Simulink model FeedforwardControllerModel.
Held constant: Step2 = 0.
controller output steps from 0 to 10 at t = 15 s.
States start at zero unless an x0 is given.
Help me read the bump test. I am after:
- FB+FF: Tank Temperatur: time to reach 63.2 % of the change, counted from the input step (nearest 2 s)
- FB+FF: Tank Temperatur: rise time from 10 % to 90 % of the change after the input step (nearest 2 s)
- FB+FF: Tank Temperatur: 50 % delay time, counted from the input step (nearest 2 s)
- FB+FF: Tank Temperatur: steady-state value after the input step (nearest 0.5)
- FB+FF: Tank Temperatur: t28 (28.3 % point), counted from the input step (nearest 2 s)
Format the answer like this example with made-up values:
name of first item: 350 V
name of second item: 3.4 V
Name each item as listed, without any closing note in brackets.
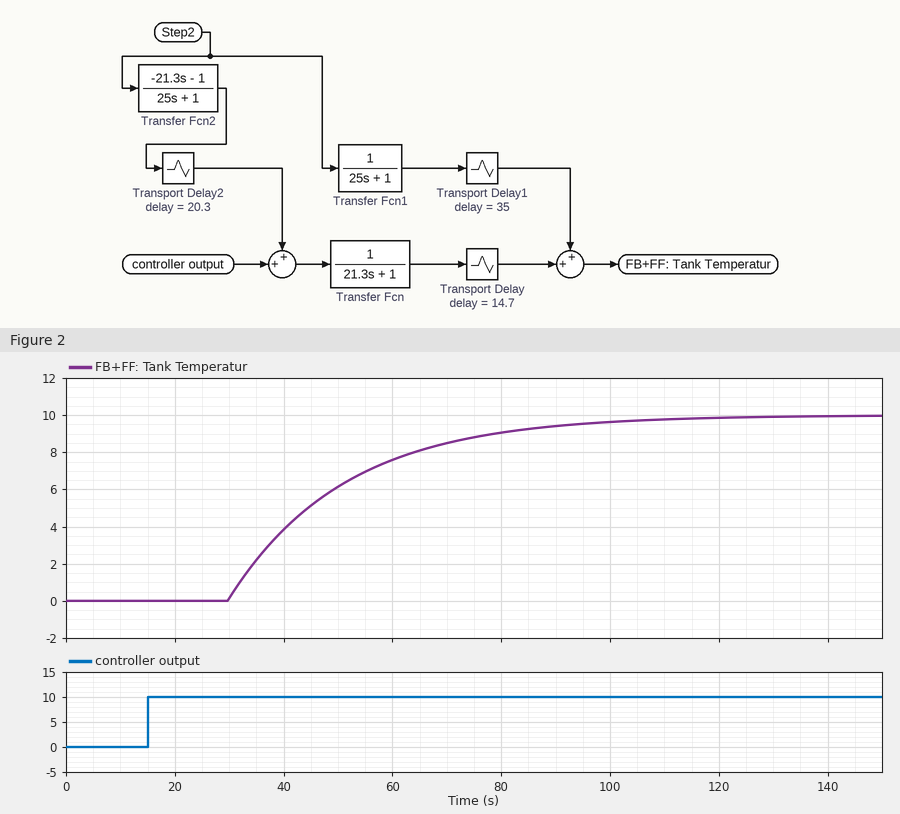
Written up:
FB+FF: Tank Temperatur: time to reach 63.2 % of the change, counted from the input step: 36 s
FB+FF: Tank Temperatur: rise time from 10 % to 90 % of the change after the input step: 46 s
FB+FF: Tank Temperatur: 50 % delay time, counted from the input step: 30 s
FB+FF: Tank Temperatur: steady-state value after the input step: 10.0
FB+FF: Tank Temperatur: t28 (28.3 % point), counted from the input step: 22 s
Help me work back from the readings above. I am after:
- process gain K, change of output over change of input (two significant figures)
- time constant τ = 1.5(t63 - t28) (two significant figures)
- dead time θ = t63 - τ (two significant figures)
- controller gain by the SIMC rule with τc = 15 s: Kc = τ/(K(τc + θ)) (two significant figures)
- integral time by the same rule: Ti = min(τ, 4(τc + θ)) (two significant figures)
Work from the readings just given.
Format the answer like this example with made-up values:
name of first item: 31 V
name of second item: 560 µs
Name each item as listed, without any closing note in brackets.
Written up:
process gain K, change of output over change of input: 1.0
time constant τ = 1.5(t63 - t28): 21 s
dead time θ = t63 - τ: 15 s
controller gain by the SIMC rule with τc = 15 s: Kc = τ/(K(τc + θ)): 0.70
integral time by the same rule: Ti = min(τ, 4(τc + θ)): 21 s
